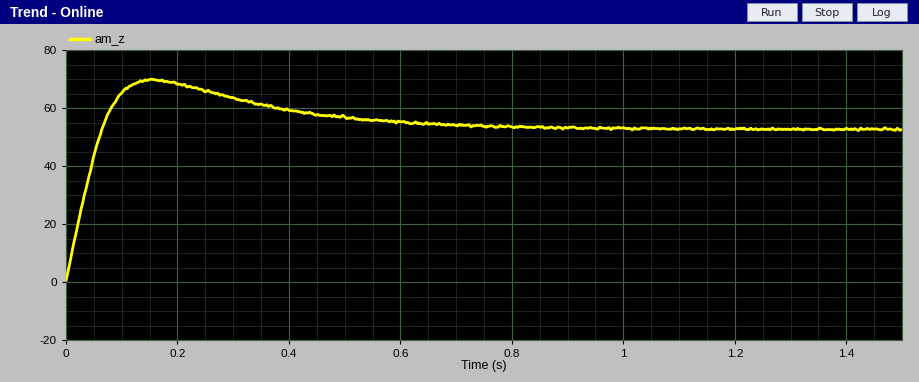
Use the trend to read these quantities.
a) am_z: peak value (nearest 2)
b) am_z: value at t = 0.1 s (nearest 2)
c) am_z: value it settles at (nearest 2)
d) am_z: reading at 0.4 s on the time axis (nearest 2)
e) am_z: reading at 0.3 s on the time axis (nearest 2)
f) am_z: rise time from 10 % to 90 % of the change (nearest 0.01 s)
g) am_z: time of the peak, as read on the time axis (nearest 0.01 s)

70
66
52
60
64
0.05 s
0.16 s
